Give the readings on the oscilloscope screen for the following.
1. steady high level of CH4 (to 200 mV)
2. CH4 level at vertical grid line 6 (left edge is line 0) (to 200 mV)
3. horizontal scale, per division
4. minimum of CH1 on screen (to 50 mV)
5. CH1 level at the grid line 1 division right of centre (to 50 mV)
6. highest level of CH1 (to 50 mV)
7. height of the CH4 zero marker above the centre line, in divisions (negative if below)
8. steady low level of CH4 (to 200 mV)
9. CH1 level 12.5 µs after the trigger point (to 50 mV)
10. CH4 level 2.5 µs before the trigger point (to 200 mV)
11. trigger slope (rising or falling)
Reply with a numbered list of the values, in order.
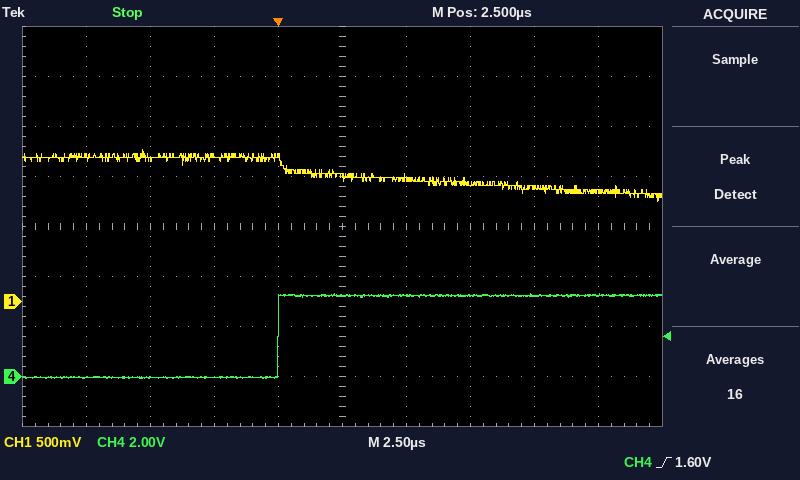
1. 3.2 V
2. 3.2 V
3. 2.5 µs
4. 1.00 V
5. 1.25 V
6. 1.50 V
7. -3.0 div
8. 0.0 V
9. 1.10 V
10. 0.0 V
11. rising
